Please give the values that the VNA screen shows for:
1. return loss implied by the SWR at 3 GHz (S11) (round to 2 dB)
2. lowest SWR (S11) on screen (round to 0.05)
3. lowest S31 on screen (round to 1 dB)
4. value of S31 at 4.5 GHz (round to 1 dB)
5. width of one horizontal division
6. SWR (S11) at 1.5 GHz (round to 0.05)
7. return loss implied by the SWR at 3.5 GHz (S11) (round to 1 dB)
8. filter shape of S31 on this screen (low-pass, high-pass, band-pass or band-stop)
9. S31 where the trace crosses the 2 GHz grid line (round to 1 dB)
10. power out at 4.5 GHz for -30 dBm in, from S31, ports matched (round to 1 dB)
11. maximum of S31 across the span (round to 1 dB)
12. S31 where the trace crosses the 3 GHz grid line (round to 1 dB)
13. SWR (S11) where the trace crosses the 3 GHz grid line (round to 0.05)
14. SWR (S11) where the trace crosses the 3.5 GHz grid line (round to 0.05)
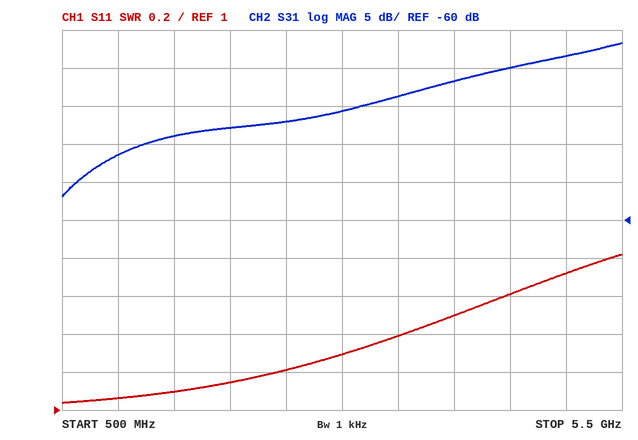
18 dB
1.05
-57 dB
-40 dB
500 MHz
1.10
16 dB
high-pass
-48 dB
-70 dBm
-37 dB
-46 dB
1.30
1.40
